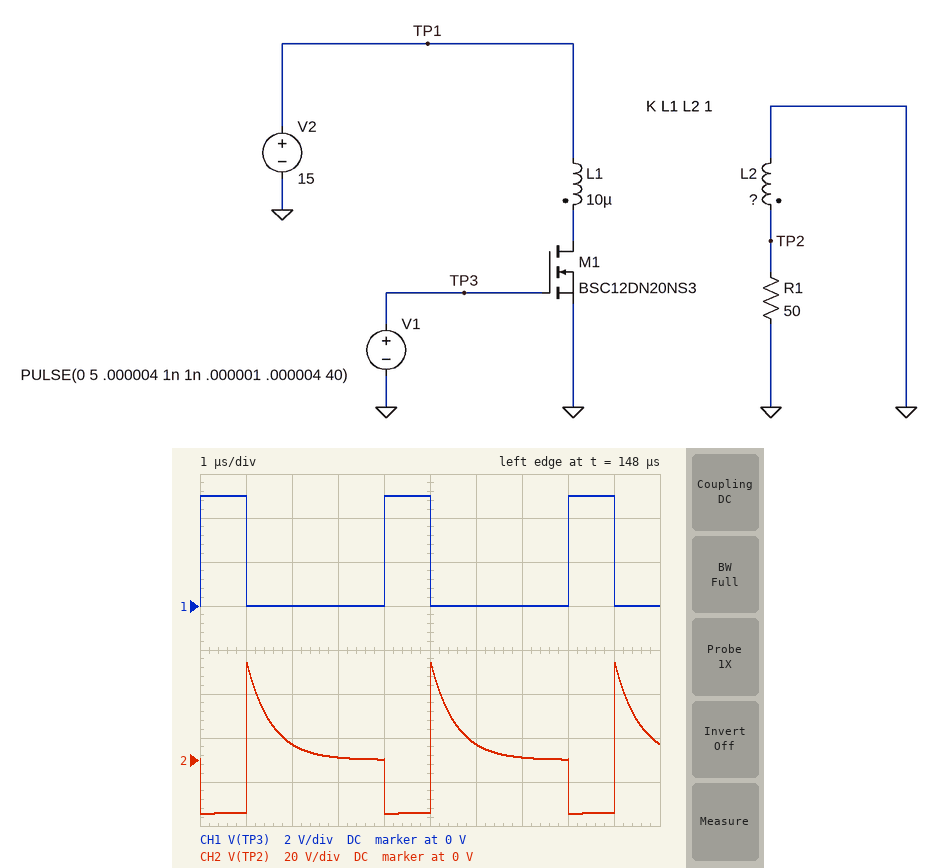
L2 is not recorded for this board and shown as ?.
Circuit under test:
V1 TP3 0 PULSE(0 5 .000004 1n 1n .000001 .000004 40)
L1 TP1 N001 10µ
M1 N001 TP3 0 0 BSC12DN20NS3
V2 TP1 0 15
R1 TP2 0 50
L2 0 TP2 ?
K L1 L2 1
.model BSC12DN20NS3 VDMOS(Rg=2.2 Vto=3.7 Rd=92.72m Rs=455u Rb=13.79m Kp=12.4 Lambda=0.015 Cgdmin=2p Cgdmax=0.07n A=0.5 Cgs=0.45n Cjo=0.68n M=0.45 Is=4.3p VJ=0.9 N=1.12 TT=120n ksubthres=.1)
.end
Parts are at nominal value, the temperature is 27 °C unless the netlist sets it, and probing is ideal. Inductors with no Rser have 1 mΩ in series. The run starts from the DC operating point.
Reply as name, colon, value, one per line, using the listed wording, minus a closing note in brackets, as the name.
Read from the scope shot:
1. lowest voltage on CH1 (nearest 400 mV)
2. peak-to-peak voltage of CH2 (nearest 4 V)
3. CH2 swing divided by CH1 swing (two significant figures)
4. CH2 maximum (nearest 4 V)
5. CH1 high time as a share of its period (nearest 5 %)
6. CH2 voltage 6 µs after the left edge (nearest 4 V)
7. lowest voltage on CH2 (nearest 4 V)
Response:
lowest voltage on CH1: 0 V
peak-to-peak voltage of CH2: 68 V
CH2 swing divided by CH1 swing: 14
CH2 maximum: 44 V
CH1 high time as a share of its period: 25 %
CH2 voltage 6 µs after the left edge: 8 V
lowest voltage on CH2: -24 V
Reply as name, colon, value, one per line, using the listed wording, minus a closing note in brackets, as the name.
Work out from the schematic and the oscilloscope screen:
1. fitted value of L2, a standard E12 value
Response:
fitted value of L2, a standard E12 value: 27 µH
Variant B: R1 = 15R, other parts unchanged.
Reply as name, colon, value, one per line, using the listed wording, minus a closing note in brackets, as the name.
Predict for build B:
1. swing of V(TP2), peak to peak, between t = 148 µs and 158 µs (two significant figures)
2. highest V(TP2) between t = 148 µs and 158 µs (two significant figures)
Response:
swing of V(TP2), peak to peak, between t = 148 µs and 158 µs: 40 V
highest V(TP2) between t = 148 µs and 158 µs: 16 V
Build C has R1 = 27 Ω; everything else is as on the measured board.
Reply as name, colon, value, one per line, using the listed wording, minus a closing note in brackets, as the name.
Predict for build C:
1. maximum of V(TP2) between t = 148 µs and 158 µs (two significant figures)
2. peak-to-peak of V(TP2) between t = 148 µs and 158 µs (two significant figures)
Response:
maximum of V(TP2) between t = 148 µs and 158 µs: 25 V
peak-to-peak of V(TP2) between t = 148 µs and 158 µs: 49 V
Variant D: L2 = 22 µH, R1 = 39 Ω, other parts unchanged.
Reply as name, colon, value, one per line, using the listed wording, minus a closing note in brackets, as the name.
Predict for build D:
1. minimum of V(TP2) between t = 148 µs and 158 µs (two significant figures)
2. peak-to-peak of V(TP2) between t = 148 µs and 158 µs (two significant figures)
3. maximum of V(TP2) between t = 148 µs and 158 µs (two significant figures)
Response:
minimum of V(TP2) between t = 148 µs and 158 µs: -22 V
peak-to-peak of V(TP2) between t = 148 µs and 158 µs: 60 V
maximum of V(TP2) between t = 148 µs and 158 µs: 38 V
